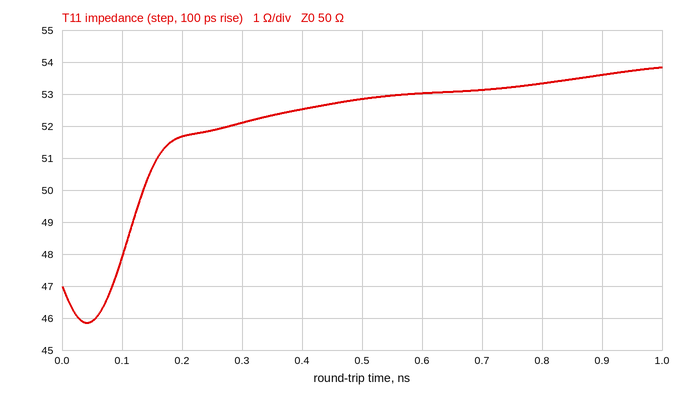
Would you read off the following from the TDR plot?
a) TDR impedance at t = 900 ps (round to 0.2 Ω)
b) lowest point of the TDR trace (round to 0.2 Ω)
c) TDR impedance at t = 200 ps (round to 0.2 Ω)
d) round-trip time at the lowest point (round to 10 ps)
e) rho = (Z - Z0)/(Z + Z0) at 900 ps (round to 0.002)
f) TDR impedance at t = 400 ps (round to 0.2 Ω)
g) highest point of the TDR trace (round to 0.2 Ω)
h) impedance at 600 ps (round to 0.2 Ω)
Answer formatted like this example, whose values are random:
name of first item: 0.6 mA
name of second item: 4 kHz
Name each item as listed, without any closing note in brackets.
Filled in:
TDR impedance at t = 900 ps: 53.6 Ω
lowest point of the TDR trace: 45.8 Ω
TDR impedance at t = 200 ps: 51.6 Ω
round-trip time at the lowest point: 40 ps
rho = (Z - Z0)/(Z + Z0) at 900 ps: +0.034
TDR impedance at t = 400 ps: 52.6 Ω
highest point of the TDR trace: 53.8 Ω
impedance at 600 ps: 53.0 Ω
